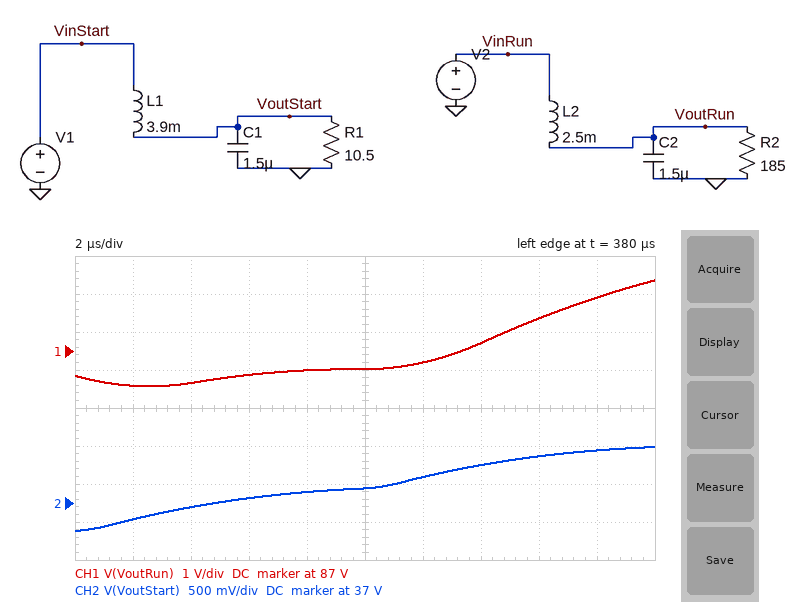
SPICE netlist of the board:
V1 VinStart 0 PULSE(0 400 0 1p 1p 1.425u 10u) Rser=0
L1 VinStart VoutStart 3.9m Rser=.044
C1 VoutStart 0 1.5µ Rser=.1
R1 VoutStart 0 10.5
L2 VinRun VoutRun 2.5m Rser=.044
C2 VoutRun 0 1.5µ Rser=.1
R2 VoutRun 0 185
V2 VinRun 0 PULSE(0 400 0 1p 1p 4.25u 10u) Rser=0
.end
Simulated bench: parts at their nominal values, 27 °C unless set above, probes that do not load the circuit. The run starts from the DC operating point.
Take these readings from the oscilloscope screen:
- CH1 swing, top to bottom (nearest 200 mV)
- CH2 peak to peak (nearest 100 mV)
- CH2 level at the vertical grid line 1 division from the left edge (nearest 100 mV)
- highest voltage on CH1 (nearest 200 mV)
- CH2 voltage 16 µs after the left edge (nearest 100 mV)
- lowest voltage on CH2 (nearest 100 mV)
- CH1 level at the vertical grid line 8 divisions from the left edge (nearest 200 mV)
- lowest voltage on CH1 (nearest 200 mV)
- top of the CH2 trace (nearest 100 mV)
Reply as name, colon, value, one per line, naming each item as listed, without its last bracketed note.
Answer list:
CH1 swing, top to bottom: 2.8 V
CH2 peak to peak: 1.1 V
CH2 level at the vertical grid line 1 division from the left edge: 36.8 V
highest voltage on CH1: 88.8 V
CH2 voltage 16 µs after the left edge: 37.6 V
lowest voltage on CH2: 36.6 V
CH1 level at the vertical grid line 8 divisions from the left edge: 87.8 V
lowest voltage on CH1: 86.0 V
top of the CH2 trace: 37.7 V
